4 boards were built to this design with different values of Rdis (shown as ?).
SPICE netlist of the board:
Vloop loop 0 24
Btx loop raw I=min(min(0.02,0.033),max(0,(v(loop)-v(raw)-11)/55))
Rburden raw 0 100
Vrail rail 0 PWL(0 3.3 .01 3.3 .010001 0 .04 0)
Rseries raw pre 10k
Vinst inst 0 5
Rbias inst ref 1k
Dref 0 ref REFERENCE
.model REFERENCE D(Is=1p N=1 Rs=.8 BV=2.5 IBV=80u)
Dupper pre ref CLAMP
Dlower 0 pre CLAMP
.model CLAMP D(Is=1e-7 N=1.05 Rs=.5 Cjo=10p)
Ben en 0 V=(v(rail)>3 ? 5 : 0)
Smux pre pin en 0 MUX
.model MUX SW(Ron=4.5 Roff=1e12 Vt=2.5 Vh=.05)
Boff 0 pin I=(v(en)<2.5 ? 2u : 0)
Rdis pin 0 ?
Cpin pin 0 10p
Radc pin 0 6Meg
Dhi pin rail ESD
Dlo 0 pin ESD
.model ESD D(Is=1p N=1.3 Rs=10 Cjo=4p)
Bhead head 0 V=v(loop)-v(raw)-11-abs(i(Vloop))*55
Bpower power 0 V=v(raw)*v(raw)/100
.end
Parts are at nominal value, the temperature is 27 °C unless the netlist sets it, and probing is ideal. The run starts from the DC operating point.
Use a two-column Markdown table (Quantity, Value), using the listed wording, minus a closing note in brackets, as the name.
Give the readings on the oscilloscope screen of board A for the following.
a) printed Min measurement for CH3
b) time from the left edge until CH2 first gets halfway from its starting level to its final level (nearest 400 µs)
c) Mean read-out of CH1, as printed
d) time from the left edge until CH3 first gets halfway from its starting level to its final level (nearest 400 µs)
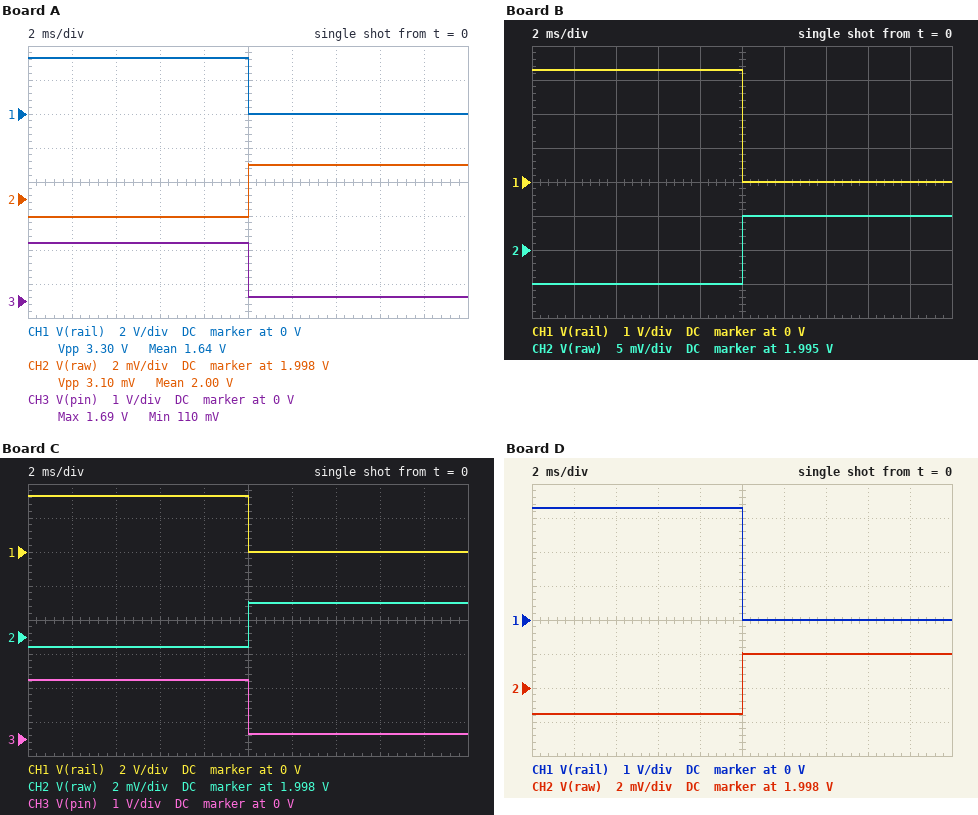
| Quantity | Value |
|---|---|
| printed Min measurement for CH3 | 110 mV |
| time from the left edge until CH2 first gets halfway from its starting level to its final level | 10.0 ms |
| Mean read-out of CH1, as printed | 1.64 V |
| time from the left edge until CH3 first gets halfway from its starting level to its final level | 10.0 ms |
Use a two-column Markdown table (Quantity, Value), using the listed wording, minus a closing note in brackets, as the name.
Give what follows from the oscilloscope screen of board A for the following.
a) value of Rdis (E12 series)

| Quantity | Value |
|---|---|
| value of Rdis | 56 kΩ |
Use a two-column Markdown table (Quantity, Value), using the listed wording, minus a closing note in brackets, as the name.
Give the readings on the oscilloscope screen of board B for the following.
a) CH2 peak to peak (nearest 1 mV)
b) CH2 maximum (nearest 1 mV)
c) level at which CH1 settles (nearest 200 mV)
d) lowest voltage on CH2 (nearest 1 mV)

| Quantity | Value |
|---|---|
| CH2 peak to peak | 10 mV |
| CH2 maximum | 2.000 V |
| level at which CH1 settles | 0 V |
| lowest voltage on CH2 | 1.990 V |
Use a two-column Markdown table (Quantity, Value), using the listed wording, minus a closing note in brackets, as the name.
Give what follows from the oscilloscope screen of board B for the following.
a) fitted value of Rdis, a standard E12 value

| Quantity | Value |
|---|---|
| fitted value of Rdis, a standard E12 value | 10 kΩ |
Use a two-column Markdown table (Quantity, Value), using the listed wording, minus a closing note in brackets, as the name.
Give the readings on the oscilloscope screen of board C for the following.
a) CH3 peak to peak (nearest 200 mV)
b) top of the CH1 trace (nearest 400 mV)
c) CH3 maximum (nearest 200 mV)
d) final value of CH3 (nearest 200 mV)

| Quantity | Value |
|---|---|
| CH3 peak to peak | 1.6 V |
| top of the CH1 trace | 3.2 V |
| CH3 maximum | 1.8 V |
| final value of CH3 | 200 mV |
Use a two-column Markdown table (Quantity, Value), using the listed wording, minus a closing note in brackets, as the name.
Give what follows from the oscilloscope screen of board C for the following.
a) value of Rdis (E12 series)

| Quantity | Value |
|---|---|
| value of Rdis | 68 kΩ |
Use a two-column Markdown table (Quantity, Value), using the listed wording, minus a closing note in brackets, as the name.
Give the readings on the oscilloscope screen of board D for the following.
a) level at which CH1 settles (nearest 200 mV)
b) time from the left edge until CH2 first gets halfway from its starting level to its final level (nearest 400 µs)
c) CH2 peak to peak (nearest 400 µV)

| Quantity | Value |
|---|---|
| level at which CH1 settles | 0 V |
| time from the left edge until CH2 first gets halfway from its starting level to its final level | 10.0 ms |
| CH2 peak to peak | 3.6 mV |
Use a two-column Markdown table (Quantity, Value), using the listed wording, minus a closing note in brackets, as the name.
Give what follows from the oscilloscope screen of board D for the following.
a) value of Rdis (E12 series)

| Quantity | Value |
|---|---|
| value of Rdis | 47 kΩ |
